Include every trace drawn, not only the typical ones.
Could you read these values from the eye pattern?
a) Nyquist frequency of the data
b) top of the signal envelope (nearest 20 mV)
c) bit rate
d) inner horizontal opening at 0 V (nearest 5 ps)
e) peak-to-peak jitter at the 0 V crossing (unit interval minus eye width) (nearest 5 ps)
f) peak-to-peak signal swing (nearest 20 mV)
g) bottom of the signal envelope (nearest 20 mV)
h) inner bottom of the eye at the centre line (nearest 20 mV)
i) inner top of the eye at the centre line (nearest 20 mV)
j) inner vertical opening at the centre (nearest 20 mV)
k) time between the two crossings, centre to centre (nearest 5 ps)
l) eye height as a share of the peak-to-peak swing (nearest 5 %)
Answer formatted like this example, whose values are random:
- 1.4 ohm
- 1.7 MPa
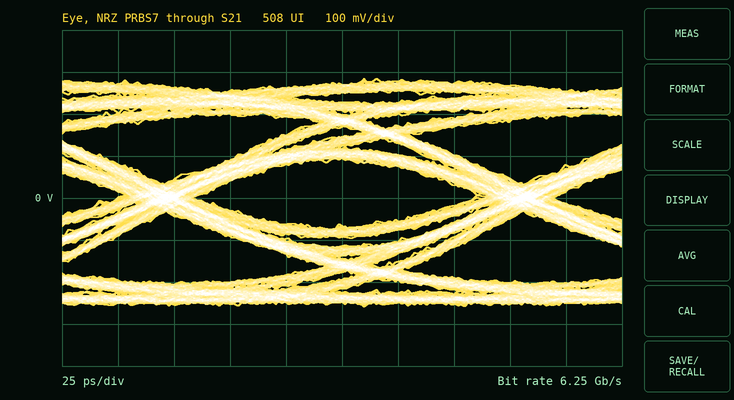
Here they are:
- 3.125 GHz
- 280 mV
- 6.25 Gb/s
- 125 ps
- 35 ps
- 540 mV
- -260 mV
- -60 mV
- 100 mV
- 160 mV
- 160 ps
- 30 %
